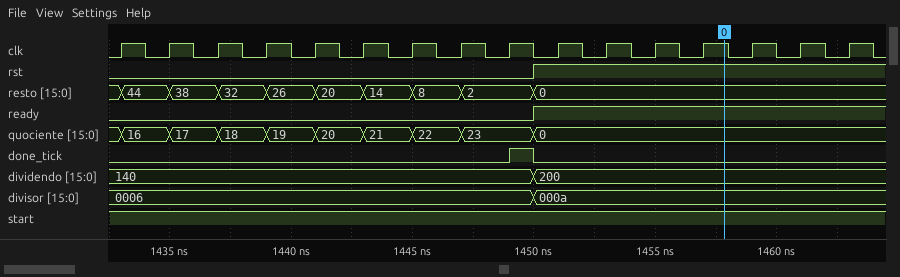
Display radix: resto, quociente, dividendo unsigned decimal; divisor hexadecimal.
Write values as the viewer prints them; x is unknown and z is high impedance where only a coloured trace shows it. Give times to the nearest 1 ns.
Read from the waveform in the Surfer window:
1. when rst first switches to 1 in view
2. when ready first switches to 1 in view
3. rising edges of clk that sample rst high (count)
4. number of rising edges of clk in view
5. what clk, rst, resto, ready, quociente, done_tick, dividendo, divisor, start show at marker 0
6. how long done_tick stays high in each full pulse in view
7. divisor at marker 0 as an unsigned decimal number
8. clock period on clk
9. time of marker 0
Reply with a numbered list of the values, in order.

1. 1450 ns
2. 1450 ns
3. 7
4. 16
5. clk=1, rst=1, resto=0, ready=1, quociente=0, done_tick=0, dividendo=200, divisor=000a, start=1
6. 1 ns
7. 10
8. 2 ns
9. 1458 ns
